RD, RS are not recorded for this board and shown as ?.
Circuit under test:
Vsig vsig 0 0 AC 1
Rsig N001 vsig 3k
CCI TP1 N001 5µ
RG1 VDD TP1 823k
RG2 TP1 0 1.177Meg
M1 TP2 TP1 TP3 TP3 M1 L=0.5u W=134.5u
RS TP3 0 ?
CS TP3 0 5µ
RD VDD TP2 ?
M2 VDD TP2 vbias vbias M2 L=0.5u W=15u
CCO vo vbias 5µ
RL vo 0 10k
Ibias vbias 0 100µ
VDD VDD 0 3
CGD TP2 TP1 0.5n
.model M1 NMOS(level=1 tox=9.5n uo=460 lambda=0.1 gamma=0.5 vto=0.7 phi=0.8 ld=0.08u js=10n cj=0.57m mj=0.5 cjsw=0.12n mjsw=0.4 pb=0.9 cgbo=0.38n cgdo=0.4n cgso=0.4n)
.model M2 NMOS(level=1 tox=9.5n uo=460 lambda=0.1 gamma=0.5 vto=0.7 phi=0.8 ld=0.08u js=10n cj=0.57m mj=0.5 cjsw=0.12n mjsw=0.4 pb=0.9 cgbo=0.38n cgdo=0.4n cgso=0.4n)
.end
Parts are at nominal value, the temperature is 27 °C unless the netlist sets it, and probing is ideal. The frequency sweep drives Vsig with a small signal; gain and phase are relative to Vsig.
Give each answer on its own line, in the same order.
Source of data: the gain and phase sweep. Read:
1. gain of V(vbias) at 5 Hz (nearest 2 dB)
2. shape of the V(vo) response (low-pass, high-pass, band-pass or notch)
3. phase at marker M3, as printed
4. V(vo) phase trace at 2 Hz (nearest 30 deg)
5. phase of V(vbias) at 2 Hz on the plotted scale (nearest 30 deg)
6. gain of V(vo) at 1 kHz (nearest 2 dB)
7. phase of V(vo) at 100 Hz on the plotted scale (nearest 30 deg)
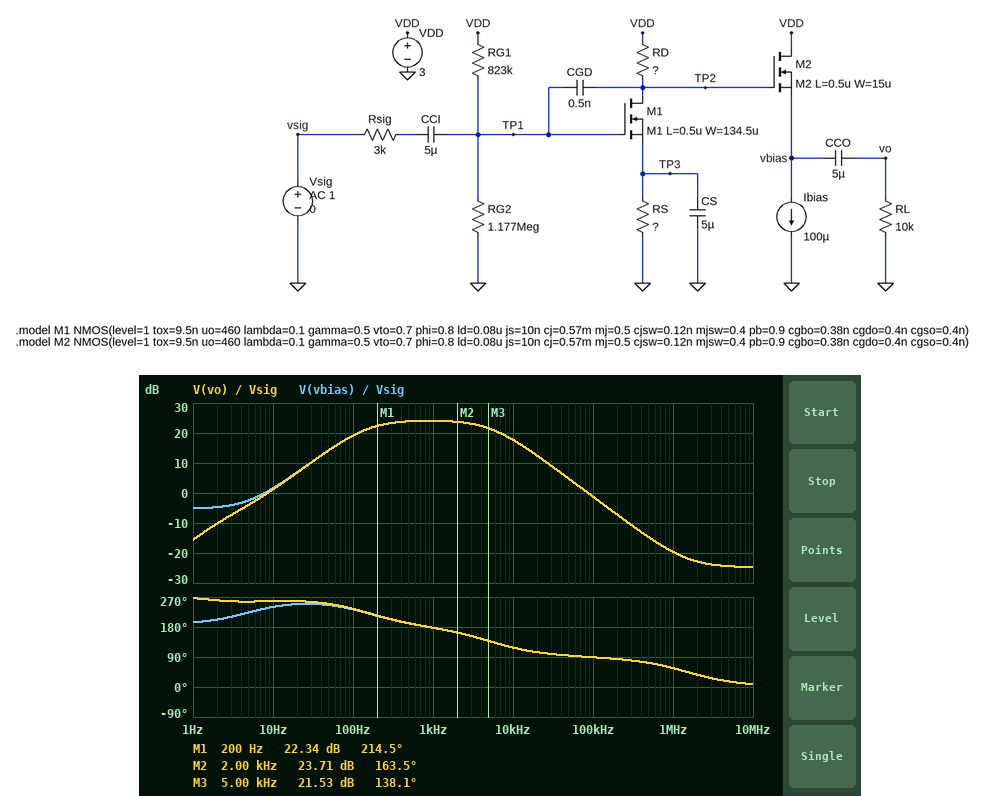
-2 dB
band-pass
138.1 deg
270 deg
210 deg
24 dB
240 deg
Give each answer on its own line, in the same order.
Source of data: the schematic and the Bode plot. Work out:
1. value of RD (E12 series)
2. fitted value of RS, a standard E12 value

3.9 kΩ
6.8 kΩ
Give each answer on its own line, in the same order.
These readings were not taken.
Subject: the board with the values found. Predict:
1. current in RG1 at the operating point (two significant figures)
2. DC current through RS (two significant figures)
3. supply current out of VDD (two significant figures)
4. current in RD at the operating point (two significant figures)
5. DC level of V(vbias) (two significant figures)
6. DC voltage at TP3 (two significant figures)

1.5 µA
150 µA
250 µA
150 µA
1.6 V
1.0 V
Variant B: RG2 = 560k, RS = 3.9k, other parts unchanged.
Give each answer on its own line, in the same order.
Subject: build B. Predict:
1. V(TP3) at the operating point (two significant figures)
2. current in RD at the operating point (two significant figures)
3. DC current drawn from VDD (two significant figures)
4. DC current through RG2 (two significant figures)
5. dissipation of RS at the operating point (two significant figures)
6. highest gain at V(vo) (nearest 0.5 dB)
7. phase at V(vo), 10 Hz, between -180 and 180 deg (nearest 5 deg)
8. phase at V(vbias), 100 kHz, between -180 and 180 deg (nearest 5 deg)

460 mV
120 µA
220 µA
2.2 µA
54 µW
23.5 dB
-115 deg
90 deg
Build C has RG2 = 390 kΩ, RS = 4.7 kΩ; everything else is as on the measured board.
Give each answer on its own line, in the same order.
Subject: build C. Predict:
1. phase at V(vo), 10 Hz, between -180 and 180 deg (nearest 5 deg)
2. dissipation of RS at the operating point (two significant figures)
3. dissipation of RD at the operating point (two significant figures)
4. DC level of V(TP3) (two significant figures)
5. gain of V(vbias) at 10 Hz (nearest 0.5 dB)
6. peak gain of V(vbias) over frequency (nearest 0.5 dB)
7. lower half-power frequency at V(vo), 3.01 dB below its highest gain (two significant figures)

-115 deg
11 µW
9.4 µW
230 mV
2.0 dB
20.0 dB
95 Hz
